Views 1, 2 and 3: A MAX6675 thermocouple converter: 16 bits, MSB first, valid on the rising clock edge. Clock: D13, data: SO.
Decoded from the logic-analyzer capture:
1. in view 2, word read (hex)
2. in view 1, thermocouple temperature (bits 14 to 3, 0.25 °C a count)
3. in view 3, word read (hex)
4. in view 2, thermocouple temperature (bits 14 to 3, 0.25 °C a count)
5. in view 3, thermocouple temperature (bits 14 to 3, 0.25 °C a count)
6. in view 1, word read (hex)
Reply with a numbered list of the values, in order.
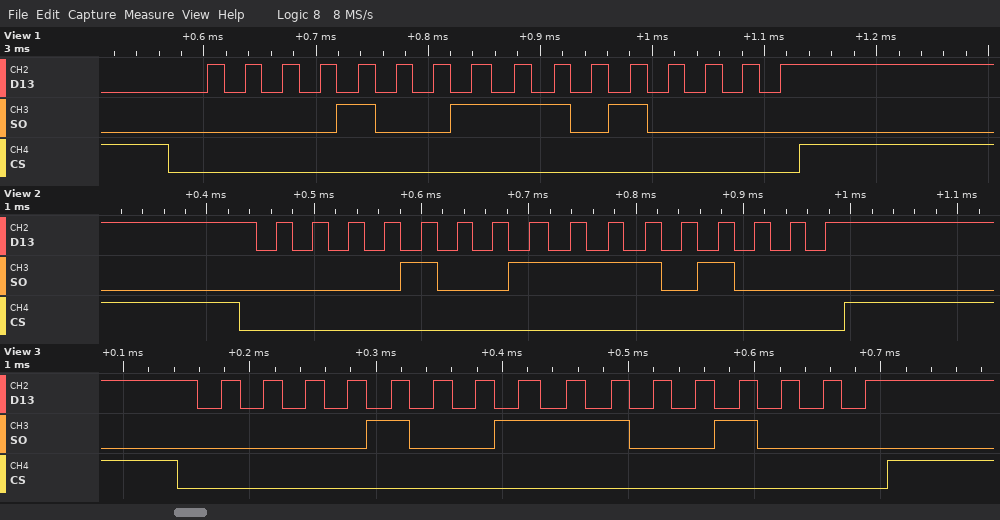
1. 0x09E8
2. 78.50 °C
3. 0x09C8
4. 79.25 °C
5. 78.25 °C
6. 0x09D0
